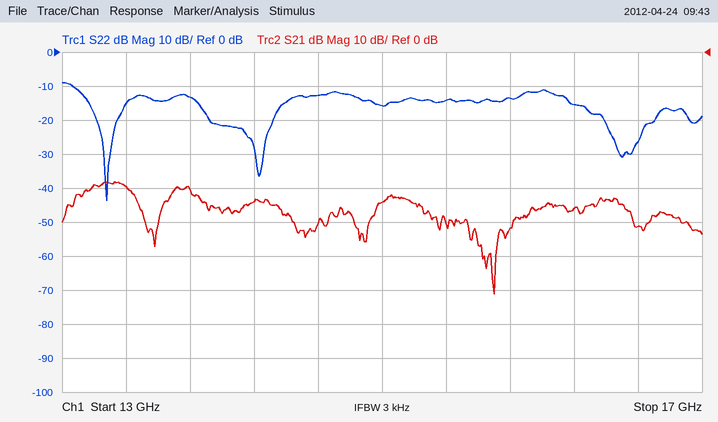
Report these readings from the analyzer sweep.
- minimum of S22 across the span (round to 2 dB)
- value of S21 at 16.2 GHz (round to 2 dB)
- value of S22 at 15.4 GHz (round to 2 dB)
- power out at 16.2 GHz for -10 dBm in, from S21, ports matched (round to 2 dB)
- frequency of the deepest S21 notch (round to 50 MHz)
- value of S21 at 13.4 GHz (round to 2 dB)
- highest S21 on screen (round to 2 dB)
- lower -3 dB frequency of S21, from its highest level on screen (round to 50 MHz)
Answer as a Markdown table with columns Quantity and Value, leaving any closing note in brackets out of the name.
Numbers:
| Quantity | Value |
|---|---|
| minimum of S22 across the span | -44 dB |
| value of S21 at 16.2 GHz | -46 dB |
| value of S22 at 15.4 GHz | -14 dB |
| power out at 16.2 GHz for -10 dBm in, from S21, ports matched | -56 dBm |
| frequency of the deepest S21 notch | 15.70 GHz |
| value of S21 at 13.4 GHz | -40 dB |
| highest S21 on screen | -38 dB |
| lower -3 dB frequency of S21, from its highest level on screen | 13.15 GHz |
